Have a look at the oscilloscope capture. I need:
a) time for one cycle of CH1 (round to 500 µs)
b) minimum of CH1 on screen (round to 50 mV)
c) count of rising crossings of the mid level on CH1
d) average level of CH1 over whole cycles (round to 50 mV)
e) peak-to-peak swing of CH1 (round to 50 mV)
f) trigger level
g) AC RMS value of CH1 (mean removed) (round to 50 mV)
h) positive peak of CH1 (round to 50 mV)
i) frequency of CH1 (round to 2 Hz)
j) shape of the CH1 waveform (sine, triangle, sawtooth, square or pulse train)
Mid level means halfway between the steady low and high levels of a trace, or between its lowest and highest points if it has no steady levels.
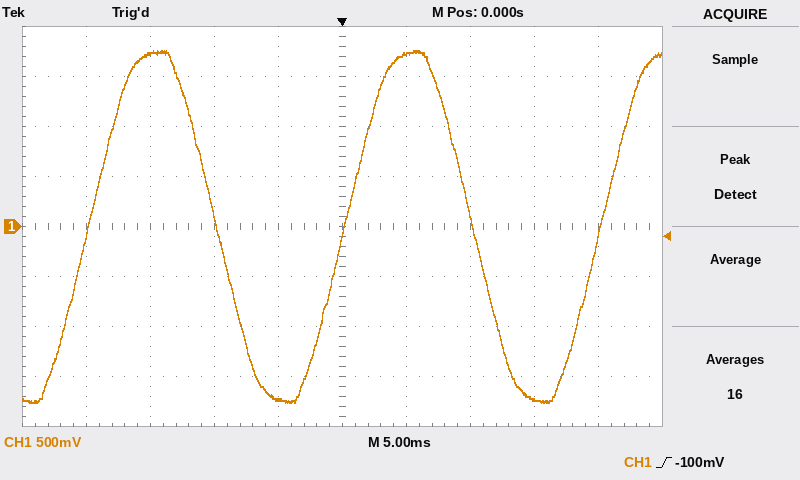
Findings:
20.0 ms
-1.75 V
3
0 mV
3.50 V
-100 mV
1.25 V
1.75 V
50 Hz
sine
